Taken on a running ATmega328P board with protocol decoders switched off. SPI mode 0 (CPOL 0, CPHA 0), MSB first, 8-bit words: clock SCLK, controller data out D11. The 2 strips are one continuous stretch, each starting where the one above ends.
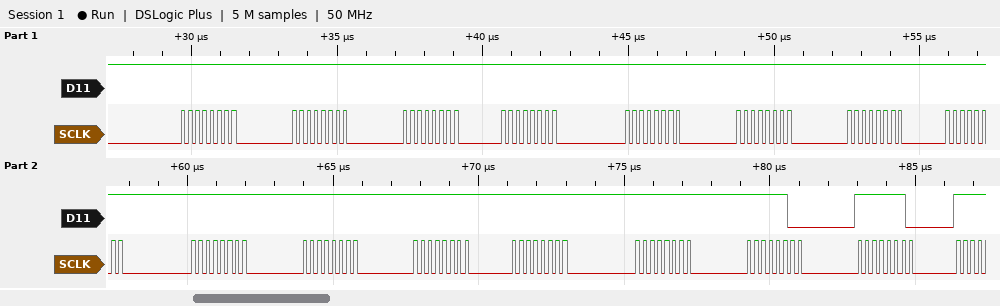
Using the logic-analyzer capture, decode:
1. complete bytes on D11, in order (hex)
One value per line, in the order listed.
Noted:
FF FF FF FF FF FF FF FF FF FF FF FF FF FC FE
